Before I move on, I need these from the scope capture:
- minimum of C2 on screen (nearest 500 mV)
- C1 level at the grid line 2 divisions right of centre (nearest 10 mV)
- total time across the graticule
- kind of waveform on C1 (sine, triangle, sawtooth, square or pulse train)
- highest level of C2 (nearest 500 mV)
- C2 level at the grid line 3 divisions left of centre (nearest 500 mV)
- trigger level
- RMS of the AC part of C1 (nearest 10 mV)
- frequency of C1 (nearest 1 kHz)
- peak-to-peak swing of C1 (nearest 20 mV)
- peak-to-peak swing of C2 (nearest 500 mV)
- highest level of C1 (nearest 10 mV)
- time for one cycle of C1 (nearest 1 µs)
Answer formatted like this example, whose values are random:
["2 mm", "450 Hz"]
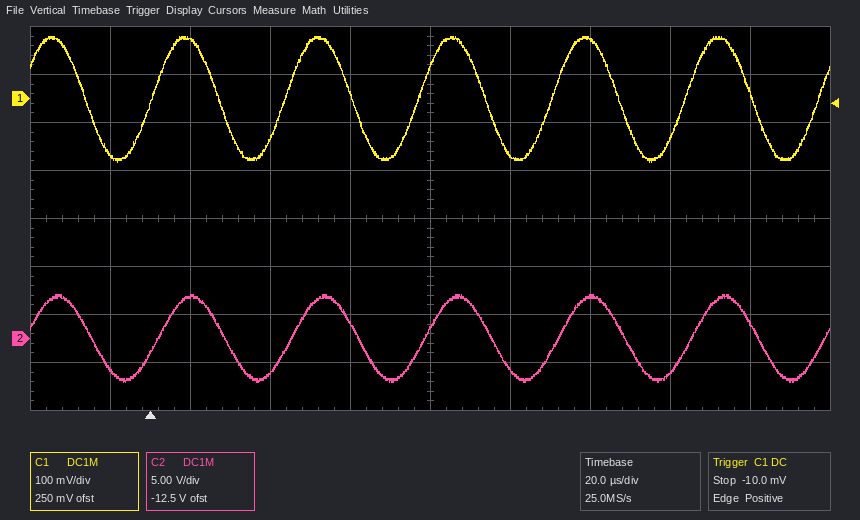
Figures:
["-4.5 V", "120 mV", "200 µs", "sine", "4.5 V", "4.5 V", "-10.0 mV", "90 mV", "30 kHz", "260 mV", "9.0 V", "130 mV", "33 µs"]
